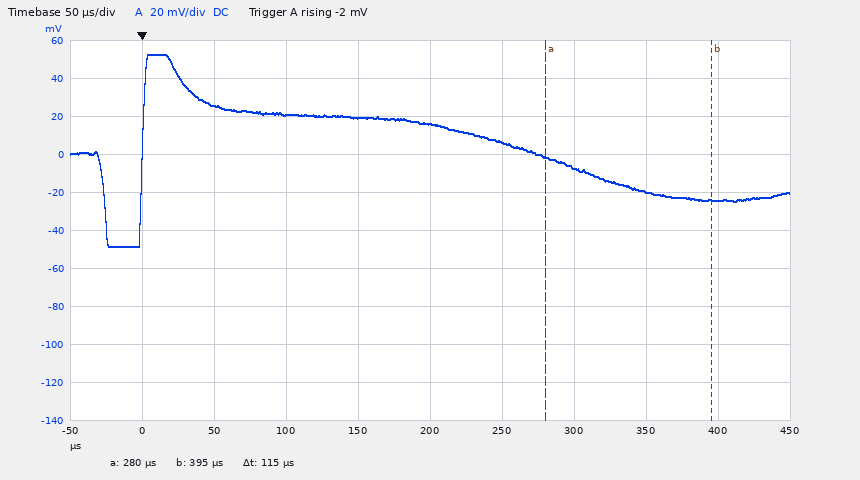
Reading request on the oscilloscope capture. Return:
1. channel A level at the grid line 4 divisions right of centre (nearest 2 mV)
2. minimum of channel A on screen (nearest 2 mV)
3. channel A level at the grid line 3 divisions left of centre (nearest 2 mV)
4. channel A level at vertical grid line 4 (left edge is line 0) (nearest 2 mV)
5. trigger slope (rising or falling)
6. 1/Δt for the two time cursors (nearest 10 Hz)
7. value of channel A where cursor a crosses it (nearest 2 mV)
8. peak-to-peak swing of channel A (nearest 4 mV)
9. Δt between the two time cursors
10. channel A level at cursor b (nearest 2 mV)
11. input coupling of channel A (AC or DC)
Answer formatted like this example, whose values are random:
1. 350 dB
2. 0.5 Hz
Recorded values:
1. -24 mV
2. -48 mV
3. 26 mV
4. 20 mV
5. rising
6. 8.70 kHz
7. -2 mV
8. 100 mV
9. 115 µs
10. -24 mV
11. DC
